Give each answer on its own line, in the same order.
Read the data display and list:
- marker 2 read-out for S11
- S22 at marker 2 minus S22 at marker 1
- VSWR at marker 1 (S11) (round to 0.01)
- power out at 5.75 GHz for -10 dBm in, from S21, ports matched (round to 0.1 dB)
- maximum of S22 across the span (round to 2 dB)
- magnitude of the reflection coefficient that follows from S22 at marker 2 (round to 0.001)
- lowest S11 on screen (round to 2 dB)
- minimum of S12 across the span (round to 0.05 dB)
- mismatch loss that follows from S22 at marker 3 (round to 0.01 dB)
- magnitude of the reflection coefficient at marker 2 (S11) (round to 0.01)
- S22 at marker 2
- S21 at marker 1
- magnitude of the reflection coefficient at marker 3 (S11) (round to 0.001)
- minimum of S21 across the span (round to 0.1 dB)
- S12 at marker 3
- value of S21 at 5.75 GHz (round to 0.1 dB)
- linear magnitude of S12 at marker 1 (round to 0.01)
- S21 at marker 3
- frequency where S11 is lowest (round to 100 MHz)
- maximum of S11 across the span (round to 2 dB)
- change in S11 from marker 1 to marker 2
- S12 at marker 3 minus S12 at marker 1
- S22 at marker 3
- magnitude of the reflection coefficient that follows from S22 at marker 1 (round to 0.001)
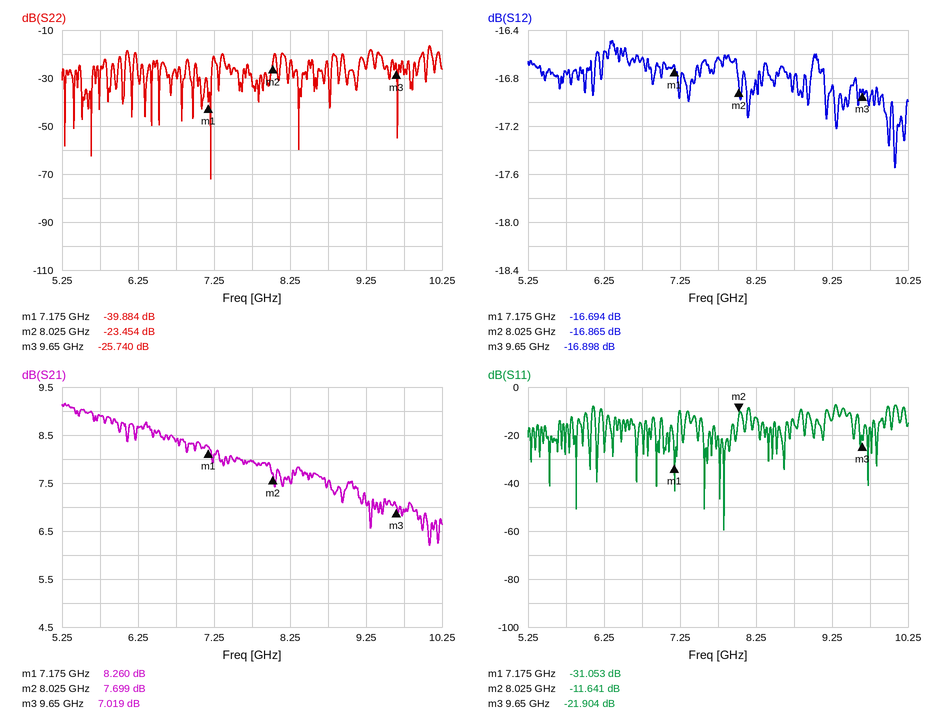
-11.641 dB
16.430 dB
1.06
-1.1 dBm
-16 dB
0.067
-60 dB
-17.55 dB
0.01 dB
0.26
-23.454 dB
8.260 dB
0.080
6.2 dB
-16.898 dB
8.9 dB
0.15
7.019 dB
7.8 GHz
-8 dB
19.412 dB
-0.204 dB
-25.740 dB
0.010
